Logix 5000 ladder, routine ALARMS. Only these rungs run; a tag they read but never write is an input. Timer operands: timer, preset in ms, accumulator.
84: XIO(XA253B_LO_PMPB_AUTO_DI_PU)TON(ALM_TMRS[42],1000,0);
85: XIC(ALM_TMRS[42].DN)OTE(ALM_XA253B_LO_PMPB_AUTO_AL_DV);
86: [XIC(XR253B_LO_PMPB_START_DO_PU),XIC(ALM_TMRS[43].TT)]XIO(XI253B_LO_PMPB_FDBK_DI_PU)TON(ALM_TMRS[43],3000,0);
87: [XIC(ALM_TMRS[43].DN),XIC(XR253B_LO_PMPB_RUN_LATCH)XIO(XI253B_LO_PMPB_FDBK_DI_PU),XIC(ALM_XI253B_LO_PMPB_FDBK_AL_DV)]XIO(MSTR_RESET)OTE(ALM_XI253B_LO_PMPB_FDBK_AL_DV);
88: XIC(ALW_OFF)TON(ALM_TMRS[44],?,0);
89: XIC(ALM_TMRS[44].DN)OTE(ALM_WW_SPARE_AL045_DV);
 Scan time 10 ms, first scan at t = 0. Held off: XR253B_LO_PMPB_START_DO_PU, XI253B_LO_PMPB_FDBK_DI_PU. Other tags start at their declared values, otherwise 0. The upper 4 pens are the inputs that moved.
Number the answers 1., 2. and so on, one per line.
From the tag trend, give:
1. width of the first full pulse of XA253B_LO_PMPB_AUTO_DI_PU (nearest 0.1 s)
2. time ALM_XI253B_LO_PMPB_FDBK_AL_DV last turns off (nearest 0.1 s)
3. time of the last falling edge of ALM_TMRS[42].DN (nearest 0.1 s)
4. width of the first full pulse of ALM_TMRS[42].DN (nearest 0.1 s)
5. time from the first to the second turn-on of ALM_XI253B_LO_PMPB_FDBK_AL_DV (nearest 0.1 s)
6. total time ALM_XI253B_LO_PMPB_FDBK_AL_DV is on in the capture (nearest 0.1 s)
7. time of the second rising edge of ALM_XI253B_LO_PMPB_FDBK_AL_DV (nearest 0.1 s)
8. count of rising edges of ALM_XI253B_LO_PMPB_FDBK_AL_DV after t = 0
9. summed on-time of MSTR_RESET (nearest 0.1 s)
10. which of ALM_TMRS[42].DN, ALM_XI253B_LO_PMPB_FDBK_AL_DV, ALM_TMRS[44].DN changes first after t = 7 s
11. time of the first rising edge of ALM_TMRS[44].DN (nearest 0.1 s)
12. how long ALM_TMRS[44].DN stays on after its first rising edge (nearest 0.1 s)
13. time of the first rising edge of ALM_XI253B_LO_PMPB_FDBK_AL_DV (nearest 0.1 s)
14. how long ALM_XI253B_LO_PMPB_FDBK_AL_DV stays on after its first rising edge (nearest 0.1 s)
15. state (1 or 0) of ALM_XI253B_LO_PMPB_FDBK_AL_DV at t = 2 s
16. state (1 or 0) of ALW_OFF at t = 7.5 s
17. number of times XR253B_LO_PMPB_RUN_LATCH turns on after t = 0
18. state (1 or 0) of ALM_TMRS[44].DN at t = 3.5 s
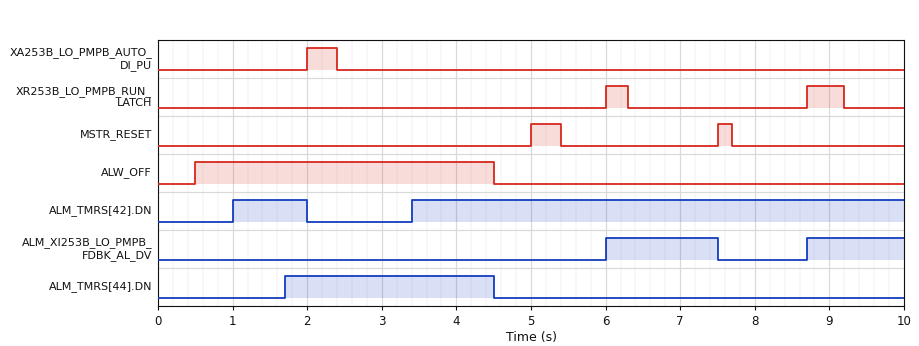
1. 0.4 s
2. 7.5 s
3. 2.0 s
4. 1.0 s
5. 2.7 s
6. 2.8 s
7. 8.7 s
8. 2
9. 0.6 s
10. ALM_XI253B_LO_PMPB_FDBK_AL_DV
11. 1.7 s
12. 2.8 s
13. 6.0 s
14. 1.5 s
15. 0
16. 0
17. 2
18. 1
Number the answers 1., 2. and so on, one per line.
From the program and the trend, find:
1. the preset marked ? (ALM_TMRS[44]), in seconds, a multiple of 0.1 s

1. 1.2 s
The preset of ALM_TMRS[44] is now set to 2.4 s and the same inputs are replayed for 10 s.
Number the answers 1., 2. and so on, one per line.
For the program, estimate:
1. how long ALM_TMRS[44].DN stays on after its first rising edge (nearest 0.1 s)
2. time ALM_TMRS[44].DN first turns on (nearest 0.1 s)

1. 1.6 s
2. 2.9 s
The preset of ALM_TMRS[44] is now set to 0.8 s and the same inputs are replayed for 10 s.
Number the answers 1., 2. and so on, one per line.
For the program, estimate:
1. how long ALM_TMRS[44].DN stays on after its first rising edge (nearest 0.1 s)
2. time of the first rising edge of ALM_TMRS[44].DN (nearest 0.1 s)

1. 3.2 s
2. 1.3 s
